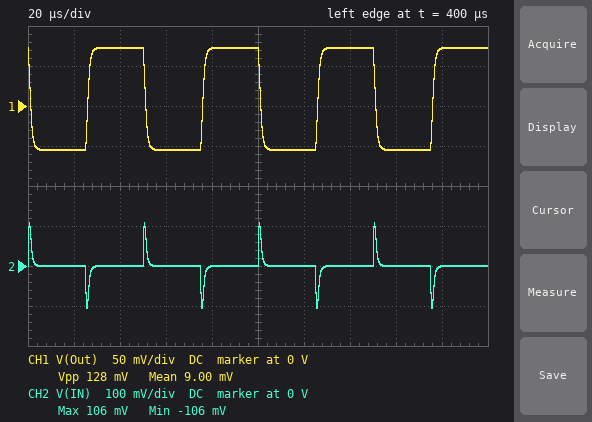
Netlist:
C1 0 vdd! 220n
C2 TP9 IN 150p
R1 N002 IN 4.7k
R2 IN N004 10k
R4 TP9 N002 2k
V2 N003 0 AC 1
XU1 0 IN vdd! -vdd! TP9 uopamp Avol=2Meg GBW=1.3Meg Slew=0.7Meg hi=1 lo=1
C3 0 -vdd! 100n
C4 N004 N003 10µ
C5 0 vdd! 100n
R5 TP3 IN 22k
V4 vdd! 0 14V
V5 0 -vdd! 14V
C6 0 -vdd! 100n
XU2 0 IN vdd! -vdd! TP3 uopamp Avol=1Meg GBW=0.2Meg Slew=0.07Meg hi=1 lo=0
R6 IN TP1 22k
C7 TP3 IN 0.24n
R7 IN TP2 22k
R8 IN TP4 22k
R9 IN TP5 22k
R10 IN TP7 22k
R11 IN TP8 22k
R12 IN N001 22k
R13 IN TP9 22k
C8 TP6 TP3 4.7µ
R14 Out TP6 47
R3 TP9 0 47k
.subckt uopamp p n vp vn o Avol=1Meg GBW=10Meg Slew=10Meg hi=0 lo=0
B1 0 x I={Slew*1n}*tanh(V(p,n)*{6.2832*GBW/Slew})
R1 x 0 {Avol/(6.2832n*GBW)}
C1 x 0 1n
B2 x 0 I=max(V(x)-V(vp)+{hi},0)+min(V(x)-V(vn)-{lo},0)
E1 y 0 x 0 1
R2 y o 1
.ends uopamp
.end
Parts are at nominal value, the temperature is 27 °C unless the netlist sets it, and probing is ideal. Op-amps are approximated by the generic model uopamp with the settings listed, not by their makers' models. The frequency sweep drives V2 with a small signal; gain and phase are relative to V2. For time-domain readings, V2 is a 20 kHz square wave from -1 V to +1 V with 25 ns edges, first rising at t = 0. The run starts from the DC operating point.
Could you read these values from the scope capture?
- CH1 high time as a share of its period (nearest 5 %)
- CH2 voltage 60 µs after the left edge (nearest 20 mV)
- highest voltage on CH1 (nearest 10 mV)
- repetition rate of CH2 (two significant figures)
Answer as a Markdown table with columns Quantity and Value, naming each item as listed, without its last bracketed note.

| Quantity | Value |
|---|---|
| CH1 high time as a share of its period | 50 % |
| CH2 voltage 60 µs after the left edge | 0 V |
| highest voltage on CH1 | 70 mV |
| repetition rate of CH2 | 20 kHz |
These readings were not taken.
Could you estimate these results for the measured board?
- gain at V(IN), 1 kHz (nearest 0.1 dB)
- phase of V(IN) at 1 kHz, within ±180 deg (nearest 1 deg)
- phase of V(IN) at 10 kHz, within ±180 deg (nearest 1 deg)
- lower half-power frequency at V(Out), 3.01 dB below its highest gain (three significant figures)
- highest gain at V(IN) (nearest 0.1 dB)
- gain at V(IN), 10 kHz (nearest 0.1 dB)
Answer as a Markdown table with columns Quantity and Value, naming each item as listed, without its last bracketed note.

| Quantity | Value |
|---|---|
| gain at V(IN), 1 kHz | -68.4 dB |
| phase of V(IN) at 1 kHz, within ±180 deg | 90 deg |
| phase of V(IN) at 10 kHz, within ±180 deg | 86 deg |
| lower half-power frequency at V(Out), 3.01 dB below its highest gain | 1.34 Hz |
| highest gain at V(IN) | -25.4 dB |
| gain at V(IN), 10 kHz | -48.4 dB |
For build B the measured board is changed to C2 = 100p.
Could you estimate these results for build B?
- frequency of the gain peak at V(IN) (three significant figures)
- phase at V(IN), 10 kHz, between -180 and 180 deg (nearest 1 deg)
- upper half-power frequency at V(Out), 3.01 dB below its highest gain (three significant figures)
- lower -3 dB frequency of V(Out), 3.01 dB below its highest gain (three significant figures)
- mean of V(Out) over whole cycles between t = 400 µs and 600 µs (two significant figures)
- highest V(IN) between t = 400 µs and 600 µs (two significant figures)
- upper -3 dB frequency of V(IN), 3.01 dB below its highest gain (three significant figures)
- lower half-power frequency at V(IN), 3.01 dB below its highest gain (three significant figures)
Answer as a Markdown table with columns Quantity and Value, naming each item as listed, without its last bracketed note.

| Quantity | Value |
|---|---|
| frequency of the gain peak at V(IN) | 350 kHz |
| phase at V(IN), 10 kHz, between -180 and 180 deg | 87 deg |
| upper half-power frequency at V(Out), 3.01 dB below its highest gain | 234 kHz |
| lower -3 dB frequency of V(Out), 3.01 dB below its highest gain | 1.34 Hz |
| mean of V(Out) over whole cycles between t = 400 µs and 600 µs | 11 mV |
| highest V(IN) between t = 400 µs and 600 µs | 140 mV |
| upper -3 dB frequency of V(IN), 3.01 dB below its highest gain | 830 kHz |
| lower half-power frequency at V(IN), 3.01 dB below its highest gain | 148 kHz |
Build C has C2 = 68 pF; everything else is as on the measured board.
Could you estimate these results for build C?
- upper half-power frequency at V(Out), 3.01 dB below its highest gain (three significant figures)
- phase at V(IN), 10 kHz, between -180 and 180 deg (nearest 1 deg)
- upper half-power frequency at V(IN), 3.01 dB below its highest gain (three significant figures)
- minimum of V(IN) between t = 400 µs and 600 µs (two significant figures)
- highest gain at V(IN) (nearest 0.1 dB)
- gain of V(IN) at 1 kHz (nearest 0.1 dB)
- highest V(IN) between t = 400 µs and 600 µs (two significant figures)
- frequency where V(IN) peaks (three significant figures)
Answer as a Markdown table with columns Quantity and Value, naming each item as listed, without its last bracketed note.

| Quantity | Value |
|---|---|
| upper half-power frequency at V(Out), 3.01 dB below its highest gain | 301 kHz |
| phase at V(IN), 10 kHz, between -180 and 180 deg | 87 deg |
| upper half-power frequency at V(IN), 3.01 dB below its highest gain | 790 kHz |
| minimum of V(IN) between t = 400 µs and 600 µs | -170 mV |
| highest gain at V(IN) | -21.6 dB |
| gain of V(IN) at 1 kHz | -68.4 dB |
| highest V(IN) between t = 400 µs and 600 µs | 170 mV |
| frequency where V(IN) peaks | 368 kHz |
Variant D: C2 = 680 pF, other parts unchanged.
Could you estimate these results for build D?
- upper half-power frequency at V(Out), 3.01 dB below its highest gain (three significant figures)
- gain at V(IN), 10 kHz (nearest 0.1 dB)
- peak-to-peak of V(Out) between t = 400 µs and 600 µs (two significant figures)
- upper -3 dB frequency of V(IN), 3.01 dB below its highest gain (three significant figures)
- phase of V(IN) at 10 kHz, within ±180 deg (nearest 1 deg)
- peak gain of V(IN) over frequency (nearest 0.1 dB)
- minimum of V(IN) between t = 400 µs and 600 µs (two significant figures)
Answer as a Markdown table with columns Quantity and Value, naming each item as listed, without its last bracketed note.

| Quantity | Value |
|---|---|
| upper half-power frequency at V(Out), 3.01 dB below its highest gain | 44.1 kHz |
| gain at V(IN), 10 kHz | -48.6 dB |
| peak-to-peak of V(Out) between t = 400 µs and 600 µs | 150 mV |
| upper -3 dB frequency of V(IN), 3.01 dB below its highest gain | 1.11 MHz |
| phase of V(IN) at 10 kHz, within ±180 deg | 77 deg |
| peak gain of V(IN) over frequency | -35.8 dB |
| minimum of V(IN) between t = 400 µs and 600 µs | -31 mV |
